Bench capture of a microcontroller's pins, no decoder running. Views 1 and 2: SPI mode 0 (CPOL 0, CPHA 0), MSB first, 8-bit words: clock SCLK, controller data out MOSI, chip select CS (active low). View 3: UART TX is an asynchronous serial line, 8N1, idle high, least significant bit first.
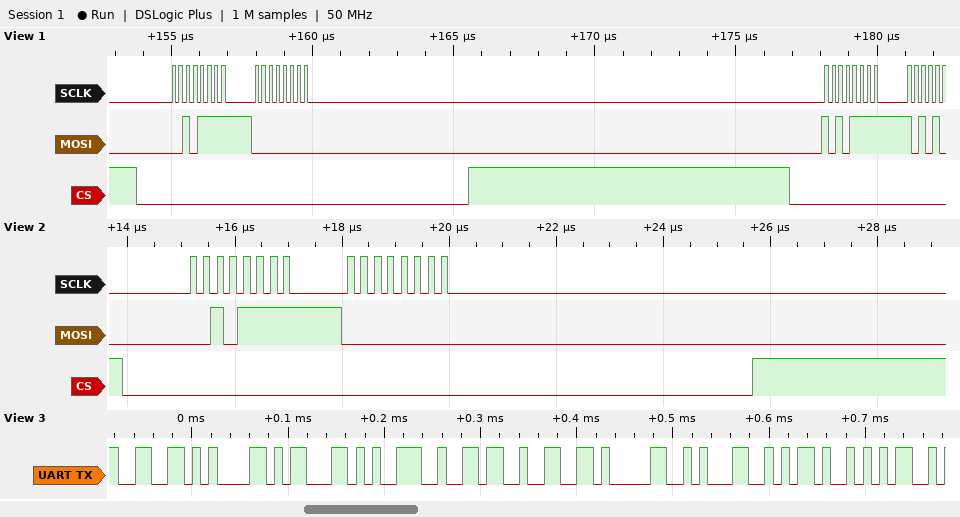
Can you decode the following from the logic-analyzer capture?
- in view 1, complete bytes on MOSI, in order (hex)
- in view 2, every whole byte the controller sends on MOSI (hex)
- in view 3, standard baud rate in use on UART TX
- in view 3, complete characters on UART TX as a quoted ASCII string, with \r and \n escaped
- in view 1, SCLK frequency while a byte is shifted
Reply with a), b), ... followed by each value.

a) 2F 00 AF
b) 2F 00
c) 115200 baud
d) "fac96f01-5"
e) 4 MHz
